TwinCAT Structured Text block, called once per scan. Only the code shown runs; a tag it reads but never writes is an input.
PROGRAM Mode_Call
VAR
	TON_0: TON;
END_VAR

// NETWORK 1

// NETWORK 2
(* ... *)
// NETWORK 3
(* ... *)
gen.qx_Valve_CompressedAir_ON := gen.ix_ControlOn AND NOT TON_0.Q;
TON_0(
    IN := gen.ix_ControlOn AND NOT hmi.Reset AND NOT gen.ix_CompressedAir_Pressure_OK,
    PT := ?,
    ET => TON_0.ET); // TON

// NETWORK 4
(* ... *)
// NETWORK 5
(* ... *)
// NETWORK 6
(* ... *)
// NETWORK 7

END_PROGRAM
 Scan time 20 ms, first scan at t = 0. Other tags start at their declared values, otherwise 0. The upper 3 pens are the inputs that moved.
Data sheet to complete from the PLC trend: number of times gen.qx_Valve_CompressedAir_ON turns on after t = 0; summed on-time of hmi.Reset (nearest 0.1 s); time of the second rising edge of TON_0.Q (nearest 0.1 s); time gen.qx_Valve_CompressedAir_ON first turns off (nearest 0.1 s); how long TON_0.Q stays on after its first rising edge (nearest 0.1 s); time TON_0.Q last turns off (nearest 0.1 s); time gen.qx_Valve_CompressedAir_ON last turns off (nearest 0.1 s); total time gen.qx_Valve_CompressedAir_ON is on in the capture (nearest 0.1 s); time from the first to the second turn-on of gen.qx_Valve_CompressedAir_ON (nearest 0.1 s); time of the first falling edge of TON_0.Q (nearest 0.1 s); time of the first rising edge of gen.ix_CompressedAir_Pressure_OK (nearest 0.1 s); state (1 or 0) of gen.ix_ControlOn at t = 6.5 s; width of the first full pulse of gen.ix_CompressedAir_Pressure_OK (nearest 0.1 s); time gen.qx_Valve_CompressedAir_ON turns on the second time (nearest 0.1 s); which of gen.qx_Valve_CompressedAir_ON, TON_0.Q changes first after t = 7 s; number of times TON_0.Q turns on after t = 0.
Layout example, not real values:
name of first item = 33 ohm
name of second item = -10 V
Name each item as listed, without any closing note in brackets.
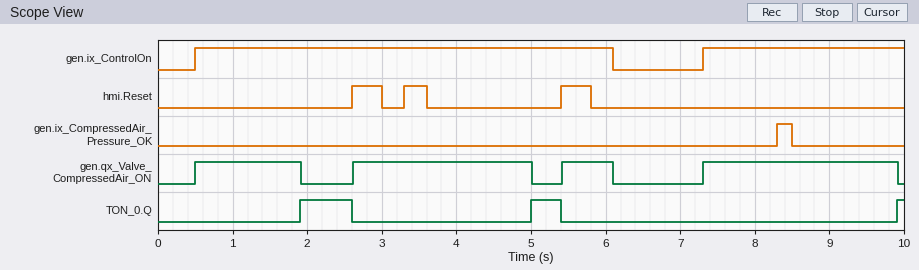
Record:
number of times gen.qx_Valve_CompressedAir_ON turns on after t = 0 = 4
summed on-time of hmi.Reset = 1.1 s
time of the second rising edge of TON_0.Q = 5.0 s
time gen.qx_Valve_CompressedAir_ON first turns off = 1.9 s
how long TON_0.Q stays on after its first rising edge = 0.7 s
time TON_0.Q last turns off = 5.4 s
time gen.qx_Valve_CompressedAir_ON last turns off = 9.9 s
total time gen.qx_Valve_CompressedAir_ON is on in the capture = 7.1 s
time from the first to the second turn-on of gen.qx_Valve_CompressedAir_ON = 2.1 s
time of the first falling edge of TON_0.Q = 2.6 s
time of the first rising edge of gen.ix_CompressedAir_Pressure_OK = 8.3 s
state (1 or 0) of gen.ix_ControlOn at t = 6.5 s = 0
width of the first full pulse of gen.ix_CompressedAir_Pressure_OK = 0.2 s
time gen.qx_Valve_CompressedAir_ON turns on the second time = 2.6 s
which of gen.qx_Valve_CompressedAir_ON, TON_0.Q changes first after t = 7 s = gen.qx_Valve_CompressedAir_ON
number of times TON_0.Q turns on after t = 0 = 3
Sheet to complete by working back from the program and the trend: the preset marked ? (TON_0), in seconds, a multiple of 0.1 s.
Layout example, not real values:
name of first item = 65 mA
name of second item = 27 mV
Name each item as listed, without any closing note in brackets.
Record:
the preset marked ? (TON_0), in seconds, a multiple of 0.1 s = 1.4 s
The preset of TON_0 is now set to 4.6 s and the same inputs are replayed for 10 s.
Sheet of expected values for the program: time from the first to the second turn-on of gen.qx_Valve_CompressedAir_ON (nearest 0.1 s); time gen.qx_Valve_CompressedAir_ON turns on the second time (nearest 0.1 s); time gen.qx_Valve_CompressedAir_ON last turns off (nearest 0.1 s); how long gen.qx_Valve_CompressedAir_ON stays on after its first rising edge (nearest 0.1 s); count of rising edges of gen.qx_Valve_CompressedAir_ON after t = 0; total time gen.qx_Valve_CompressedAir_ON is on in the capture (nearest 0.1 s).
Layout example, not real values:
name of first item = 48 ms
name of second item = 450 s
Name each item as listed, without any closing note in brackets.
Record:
time from the first to the second turn-on of gen.qx_Valve_CompressedAir_ON = 6.8 s
time gen.qx_Valve_CompressedAir_ON turns on the second time = 7.3 s
time gen.qx_Valve_CompressedAir_ON last turns off = 6.1 s
how long gen.qx_Valve_CompressedAir_ON stays on after its first rising edge = 5.6 s
count of rising edges of gen.qx_Valve_CompressedAir_ON after t = 0 = 2
total time gen.qx_Valve_CompressedAir_ON is on in the capture = 8.3 s
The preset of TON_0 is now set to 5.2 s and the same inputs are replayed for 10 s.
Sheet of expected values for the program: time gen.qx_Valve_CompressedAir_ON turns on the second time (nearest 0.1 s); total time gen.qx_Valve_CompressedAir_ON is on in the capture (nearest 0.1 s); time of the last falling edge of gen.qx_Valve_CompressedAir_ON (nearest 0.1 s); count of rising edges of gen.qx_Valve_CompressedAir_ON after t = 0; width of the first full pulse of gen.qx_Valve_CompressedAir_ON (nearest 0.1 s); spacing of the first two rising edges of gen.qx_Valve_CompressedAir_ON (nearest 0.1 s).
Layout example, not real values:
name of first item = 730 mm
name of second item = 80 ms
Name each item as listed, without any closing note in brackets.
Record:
time gen.qx_Valve_CompressedAir_ON turns on the second time = 7.3 s
total time gen.qx_Valve_CompressedAir_ON is on in the capture = 8.3 s
time of the last falling edge of gen.qx_Valve_CompressedAir_ON = 6.1 s
count of rising edges of gen.qx_Valve_CompressedAir_ON after t = 0 = 2
width of the first full pulse of gen.qx_Valve_CompressedAir_ON = 5.6 s
spacing of the first two rising edges of gen.qx_Valve_CompressedAir_ON = 6.8 s
